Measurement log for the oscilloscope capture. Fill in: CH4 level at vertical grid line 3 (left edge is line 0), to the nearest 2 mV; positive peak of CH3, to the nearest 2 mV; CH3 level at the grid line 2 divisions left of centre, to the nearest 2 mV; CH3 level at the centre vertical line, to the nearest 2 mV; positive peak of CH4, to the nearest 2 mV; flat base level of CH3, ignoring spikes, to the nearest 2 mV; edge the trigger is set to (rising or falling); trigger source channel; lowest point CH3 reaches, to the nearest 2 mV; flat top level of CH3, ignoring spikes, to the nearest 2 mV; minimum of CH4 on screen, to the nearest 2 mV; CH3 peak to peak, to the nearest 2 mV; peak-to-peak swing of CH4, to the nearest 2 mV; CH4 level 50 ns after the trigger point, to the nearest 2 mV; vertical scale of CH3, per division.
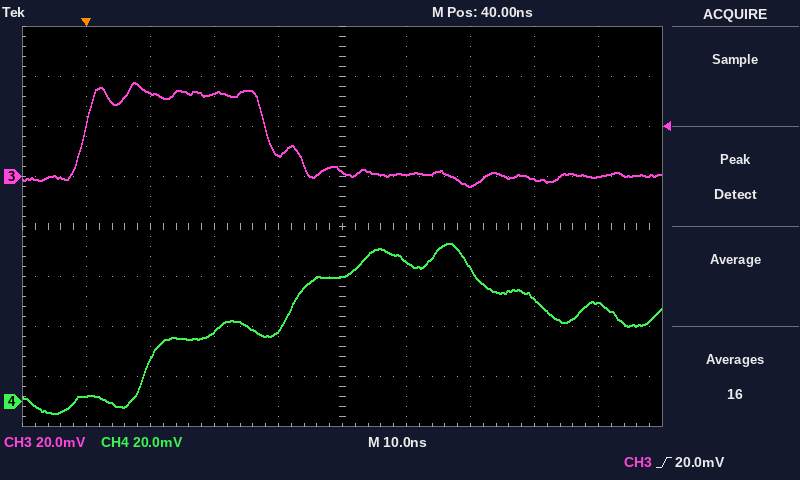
28 mV
38 mV
34 mV
2 mV
64 mV
0 mV
rising
CH3
-4 mV
34 mV
-4 mV
42 mV
68 mV
56 mV
20 mV
